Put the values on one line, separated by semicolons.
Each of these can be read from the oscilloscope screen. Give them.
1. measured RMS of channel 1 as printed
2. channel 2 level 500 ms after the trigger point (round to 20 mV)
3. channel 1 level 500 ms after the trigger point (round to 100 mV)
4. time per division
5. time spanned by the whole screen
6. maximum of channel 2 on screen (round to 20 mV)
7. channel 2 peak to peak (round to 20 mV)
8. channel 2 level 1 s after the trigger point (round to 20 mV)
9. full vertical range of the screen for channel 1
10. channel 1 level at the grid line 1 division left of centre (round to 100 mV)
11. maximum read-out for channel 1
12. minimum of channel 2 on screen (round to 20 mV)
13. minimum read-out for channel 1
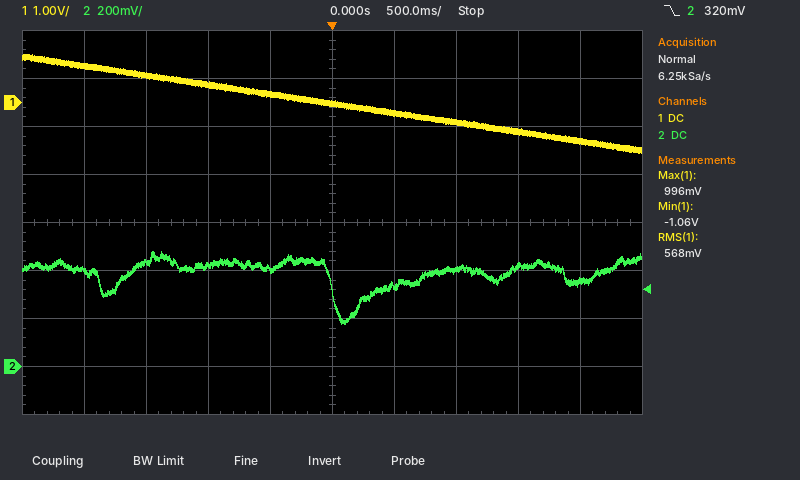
568 mV; 340 mV; -200 mV; 500 ms; 5 s; 480 mV; 300 mV; 400 mV; 8 V; 200 mV; 996 mV; 180 mV; -1.06 V
